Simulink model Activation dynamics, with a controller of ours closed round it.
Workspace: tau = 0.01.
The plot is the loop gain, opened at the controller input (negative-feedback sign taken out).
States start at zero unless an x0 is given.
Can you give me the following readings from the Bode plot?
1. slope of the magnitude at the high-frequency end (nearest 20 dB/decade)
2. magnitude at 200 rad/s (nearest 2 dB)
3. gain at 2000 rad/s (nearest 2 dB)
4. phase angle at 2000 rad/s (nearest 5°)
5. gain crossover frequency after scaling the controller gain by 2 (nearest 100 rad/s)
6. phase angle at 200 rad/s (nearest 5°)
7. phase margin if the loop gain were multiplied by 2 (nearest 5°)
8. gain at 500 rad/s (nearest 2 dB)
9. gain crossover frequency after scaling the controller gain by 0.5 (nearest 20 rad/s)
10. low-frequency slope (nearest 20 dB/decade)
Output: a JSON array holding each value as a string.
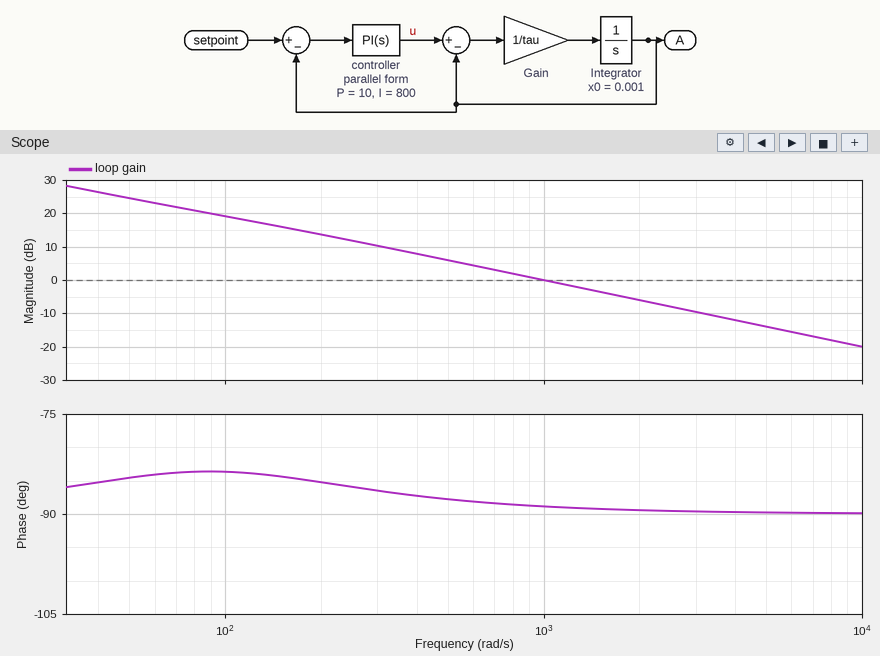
["-20 dB/decade", "14 dB", "-6 dB", "-90°", "2000 rad/s", "-85°", "90°", "6 dB", "500 rad/s", "-20 dB/decade"]
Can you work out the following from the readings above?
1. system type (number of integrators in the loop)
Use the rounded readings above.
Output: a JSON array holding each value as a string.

["1"]
